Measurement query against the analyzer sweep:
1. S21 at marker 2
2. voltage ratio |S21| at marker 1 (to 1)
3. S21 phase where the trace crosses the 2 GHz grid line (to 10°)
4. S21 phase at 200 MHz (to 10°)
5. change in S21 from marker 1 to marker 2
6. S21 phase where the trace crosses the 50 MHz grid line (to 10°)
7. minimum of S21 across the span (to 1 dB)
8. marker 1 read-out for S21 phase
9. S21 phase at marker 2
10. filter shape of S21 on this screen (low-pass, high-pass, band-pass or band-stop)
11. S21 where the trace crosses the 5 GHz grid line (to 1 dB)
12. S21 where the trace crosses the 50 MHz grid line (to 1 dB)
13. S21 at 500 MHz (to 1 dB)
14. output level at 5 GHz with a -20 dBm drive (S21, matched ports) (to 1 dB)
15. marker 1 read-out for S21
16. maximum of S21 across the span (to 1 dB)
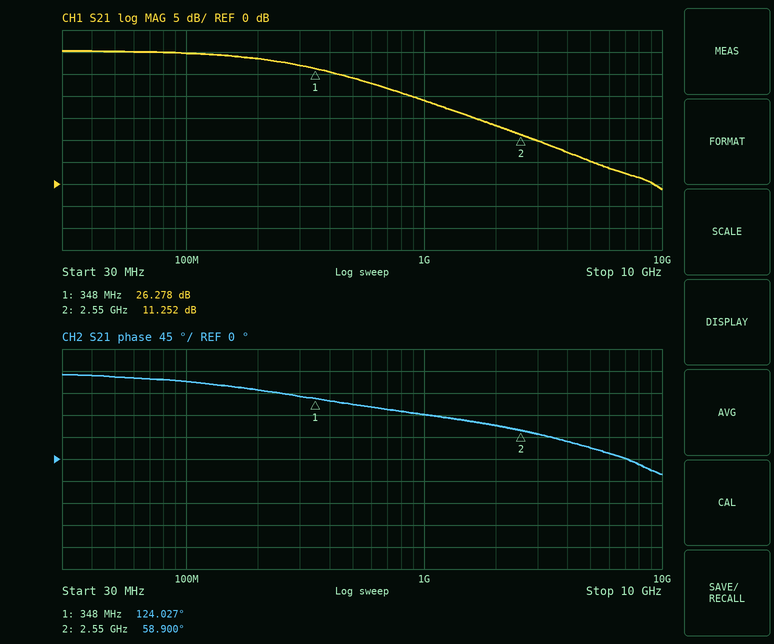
11.252 dB
21
70°
140°
-15.026 dB
170°
-1 dB
124.027°
58.900°
low-pass
5 dB
30 dB
24 dB
-15 dBm
26.278 dB
30 dB
